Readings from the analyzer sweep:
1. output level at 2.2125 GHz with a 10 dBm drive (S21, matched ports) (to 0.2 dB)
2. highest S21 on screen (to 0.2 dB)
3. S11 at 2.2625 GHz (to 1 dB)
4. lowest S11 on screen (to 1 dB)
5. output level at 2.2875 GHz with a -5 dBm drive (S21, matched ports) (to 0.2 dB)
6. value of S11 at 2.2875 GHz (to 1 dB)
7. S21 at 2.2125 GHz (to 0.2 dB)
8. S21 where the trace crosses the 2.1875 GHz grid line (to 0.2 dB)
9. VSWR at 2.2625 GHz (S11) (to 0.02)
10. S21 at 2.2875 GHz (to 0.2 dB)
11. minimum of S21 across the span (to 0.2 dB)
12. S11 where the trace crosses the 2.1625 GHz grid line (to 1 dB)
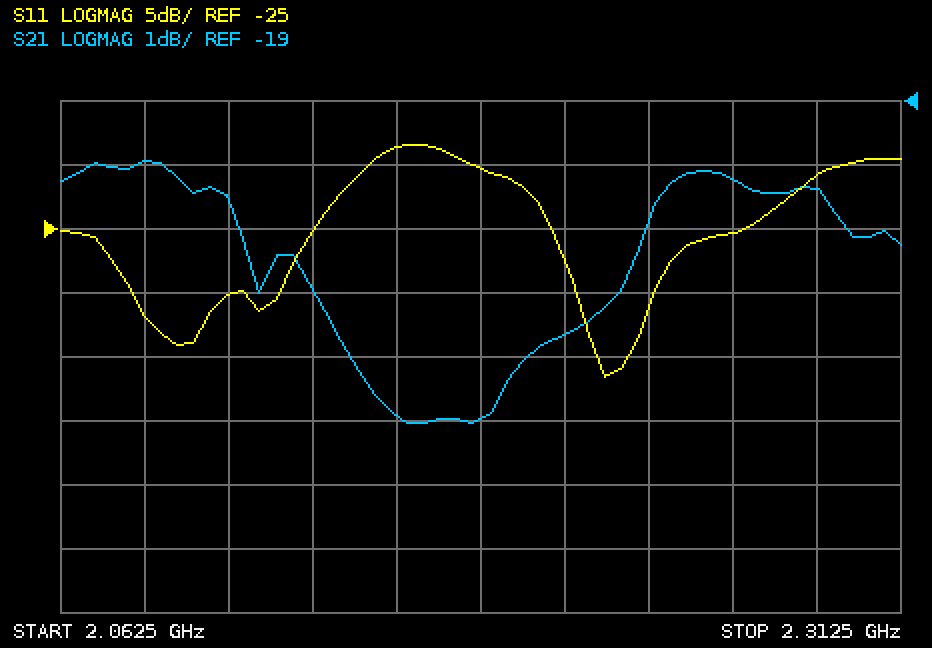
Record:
-12.6 dBm
-20.0 dB
-25 dB
-37 dB
-25.4 dBm
-21 dB
-22.6 dB
-24.0 dB
1.12
-20.4 dB
-24.0 dB
-19 dB
